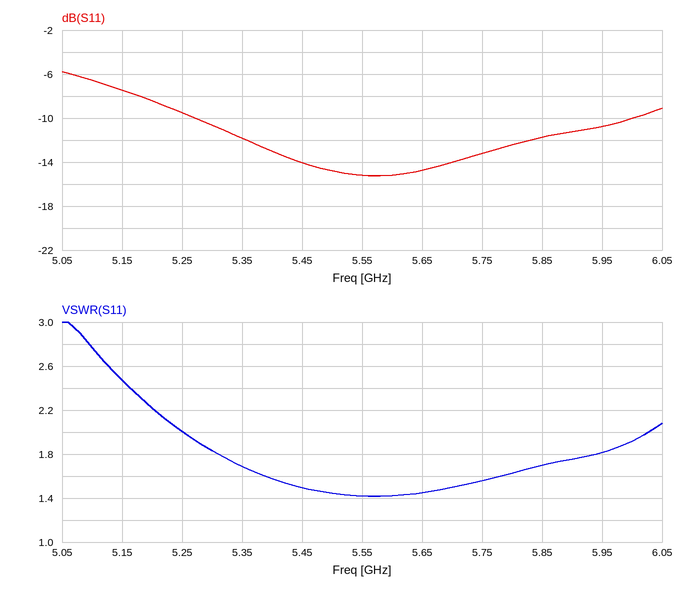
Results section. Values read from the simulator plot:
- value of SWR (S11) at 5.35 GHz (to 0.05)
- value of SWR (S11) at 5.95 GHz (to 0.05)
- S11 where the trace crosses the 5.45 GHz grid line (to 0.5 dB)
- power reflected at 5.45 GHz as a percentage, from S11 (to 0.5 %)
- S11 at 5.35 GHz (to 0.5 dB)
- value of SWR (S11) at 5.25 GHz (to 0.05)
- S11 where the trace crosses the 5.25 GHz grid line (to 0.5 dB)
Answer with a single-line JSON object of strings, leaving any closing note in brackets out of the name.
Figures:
{"value of SWR (S11) at 5.35 GHz": "1.70", "value of SWR (S11) at 5.95 GHz": "1.80", "S11 where the trace crosses the 5.45 GHz grid line": "-14.0 dB", "power reflected at 5.45 GHz as a percentage, from S11": "4.0 %", "S11 at 5.35 GHz": "-12.0 dB", "value of SWR (S11) at 5.25 GHz": "2.00", "S11 where the trace crosses the 5.25 GHz grid line": "-9.5 dB"}
